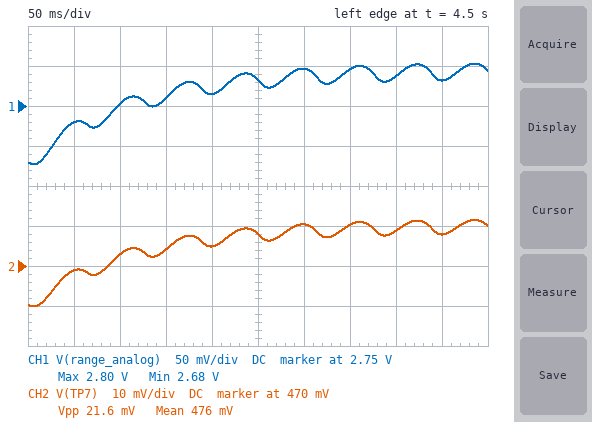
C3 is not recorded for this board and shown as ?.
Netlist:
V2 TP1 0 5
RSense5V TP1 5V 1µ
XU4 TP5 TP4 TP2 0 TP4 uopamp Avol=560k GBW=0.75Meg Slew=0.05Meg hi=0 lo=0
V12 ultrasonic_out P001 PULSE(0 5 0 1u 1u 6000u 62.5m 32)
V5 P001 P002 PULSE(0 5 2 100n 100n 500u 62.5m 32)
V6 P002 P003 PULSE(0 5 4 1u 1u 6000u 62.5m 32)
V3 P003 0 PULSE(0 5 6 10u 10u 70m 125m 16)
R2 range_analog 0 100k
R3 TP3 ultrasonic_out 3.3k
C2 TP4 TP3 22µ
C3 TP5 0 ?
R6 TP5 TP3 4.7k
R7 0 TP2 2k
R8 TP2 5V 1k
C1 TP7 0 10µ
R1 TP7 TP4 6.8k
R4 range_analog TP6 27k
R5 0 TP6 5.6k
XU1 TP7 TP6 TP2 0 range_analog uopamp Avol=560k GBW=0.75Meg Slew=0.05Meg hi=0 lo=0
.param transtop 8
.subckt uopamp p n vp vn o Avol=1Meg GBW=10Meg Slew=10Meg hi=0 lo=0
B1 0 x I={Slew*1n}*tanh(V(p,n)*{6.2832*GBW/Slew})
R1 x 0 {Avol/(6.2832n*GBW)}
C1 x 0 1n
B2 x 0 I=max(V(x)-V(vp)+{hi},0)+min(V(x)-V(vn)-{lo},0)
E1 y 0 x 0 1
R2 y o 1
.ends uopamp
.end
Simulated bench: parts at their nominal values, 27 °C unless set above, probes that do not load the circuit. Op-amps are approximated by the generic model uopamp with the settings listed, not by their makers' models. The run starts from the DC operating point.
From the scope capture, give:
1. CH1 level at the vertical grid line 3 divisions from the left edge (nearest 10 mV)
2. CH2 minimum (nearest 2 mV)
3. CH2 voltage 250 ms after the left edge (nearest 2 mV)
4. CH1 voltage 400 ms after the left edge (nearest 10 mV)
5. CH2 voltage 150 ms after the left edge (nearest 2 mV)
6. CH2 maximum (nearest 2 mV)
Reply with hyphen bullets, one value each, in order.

- 2.76 V
- 460 mV
- 478 mV
- 2.79 V
- 474 mV
- 482 mV
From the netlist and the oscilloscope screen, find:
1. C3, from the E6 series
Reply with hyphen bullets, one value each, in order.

- 22 µF
